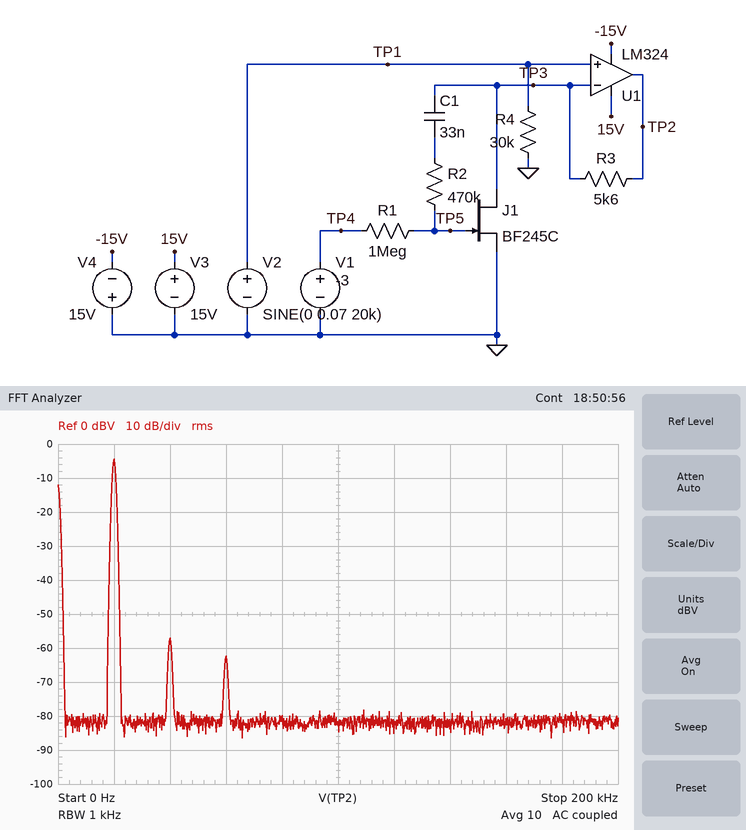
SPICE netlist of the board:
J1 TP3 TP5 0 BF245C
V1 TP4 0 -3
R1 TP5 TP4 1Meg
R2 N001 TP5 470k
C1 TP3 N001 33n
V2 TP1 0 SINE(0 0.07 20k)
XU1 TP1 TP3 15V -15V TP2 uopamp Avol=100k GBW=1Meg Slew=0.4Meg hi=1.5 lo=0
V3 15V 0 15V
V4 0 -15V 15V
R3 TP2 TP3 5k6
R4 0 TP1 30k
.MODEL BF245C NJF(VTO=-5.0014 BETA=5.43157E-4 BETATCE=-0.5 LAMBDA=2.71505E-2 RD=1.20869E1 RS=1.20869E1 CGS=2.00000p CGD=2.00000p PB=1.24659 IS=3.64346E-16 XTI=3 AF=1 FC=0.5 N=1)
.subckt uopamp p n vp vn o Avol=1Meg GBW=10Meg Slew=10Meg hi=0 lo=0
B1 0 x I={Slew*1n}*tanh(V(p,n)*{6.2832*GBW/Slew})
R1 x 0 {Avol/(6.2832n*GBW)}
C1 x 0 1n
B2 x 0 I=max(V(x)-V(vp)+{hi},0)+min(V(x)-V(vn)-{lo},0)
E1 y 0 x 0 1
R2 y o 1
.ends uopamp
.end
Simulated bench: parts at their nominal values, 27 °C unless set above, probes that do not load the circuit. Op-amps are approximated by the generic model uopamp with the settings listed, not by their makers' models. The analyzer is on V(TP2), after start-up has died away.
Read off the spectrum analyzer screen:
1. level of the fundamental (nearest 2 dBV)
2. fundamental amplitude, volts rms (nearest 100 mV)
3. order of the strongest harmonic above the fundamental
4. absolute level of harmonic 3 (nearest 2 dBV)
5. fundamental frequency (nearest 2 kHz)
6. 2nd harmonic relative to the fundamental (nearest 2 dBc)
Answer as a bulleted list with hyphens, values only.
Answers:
- -4 dBV
- 600 mV
- 2
- -62 dBV
- 20 kHz
- -52 dBc
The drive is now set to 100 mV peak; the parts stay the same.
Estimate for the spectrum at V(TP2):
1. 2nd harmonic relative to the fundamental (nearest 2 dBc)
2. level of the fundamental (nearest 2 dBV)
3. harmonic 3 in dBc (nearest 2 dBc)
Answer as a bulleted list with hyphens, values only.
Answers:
- -50 dBc
- -2 dBV
- -52 dBc
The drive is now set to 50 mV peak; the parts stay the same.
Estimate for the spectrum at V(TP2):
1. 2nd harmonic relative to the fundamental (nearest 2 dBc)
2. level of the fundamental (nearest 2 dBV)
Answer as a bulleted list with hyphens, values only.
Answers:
- -56 dBc
- -8 dBV
